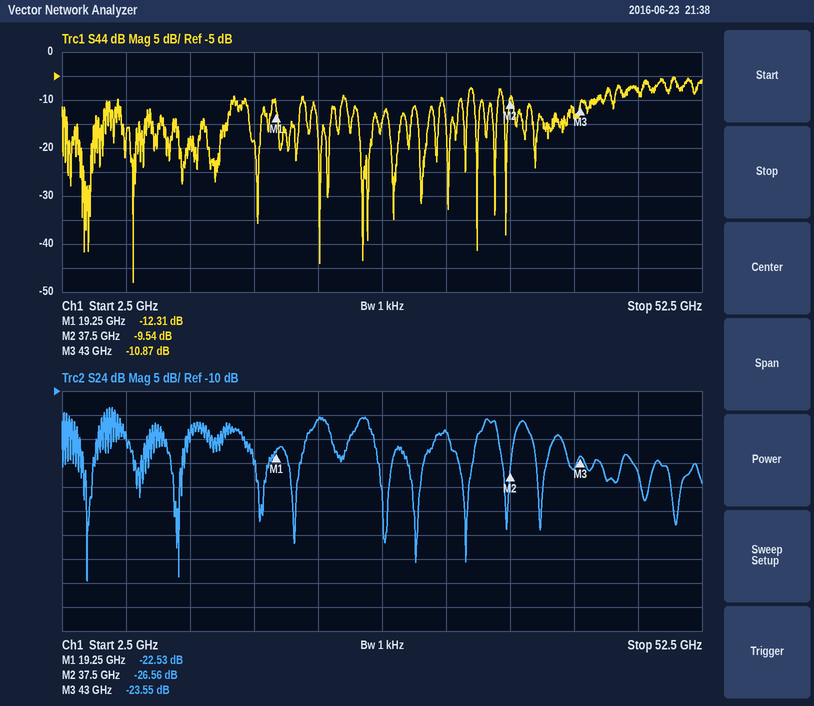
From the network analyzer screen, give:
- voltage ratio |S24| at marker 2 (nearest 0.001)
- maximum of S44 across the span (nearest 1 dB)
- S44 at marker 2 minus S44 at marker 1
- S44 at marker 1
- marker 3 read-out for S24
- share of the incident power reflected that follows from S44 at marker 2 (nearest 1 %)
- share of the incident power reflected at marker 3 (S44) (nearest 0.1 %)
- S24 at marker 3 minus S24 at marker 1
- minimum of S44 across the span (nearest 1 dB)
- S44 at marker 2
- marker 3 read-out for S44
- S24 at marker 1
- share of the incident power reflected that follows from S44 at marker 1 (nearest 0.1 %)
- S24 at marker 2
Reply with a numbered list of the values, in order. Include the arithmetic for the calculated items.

1. 10^(-26.56/20) ≈ 0.047
2. -5 dB
3. -9.54 − (-12.31) = 2.77 dB
4. -12.31 dB
5. -23.55 dB
6. 10^(-9.54/10) ≈ 11 %
7. 10^(-10.87/10) ≈ 8.2 %
8. -23.55 − (-22.53) = -1.02 dB
9. -48 dB
10. -9.54 dB
11. -10.87 dB
12. -22.53 dB
13. 10^(-12.31/10) ≈ 5.9 %
14. -26.56 dB
